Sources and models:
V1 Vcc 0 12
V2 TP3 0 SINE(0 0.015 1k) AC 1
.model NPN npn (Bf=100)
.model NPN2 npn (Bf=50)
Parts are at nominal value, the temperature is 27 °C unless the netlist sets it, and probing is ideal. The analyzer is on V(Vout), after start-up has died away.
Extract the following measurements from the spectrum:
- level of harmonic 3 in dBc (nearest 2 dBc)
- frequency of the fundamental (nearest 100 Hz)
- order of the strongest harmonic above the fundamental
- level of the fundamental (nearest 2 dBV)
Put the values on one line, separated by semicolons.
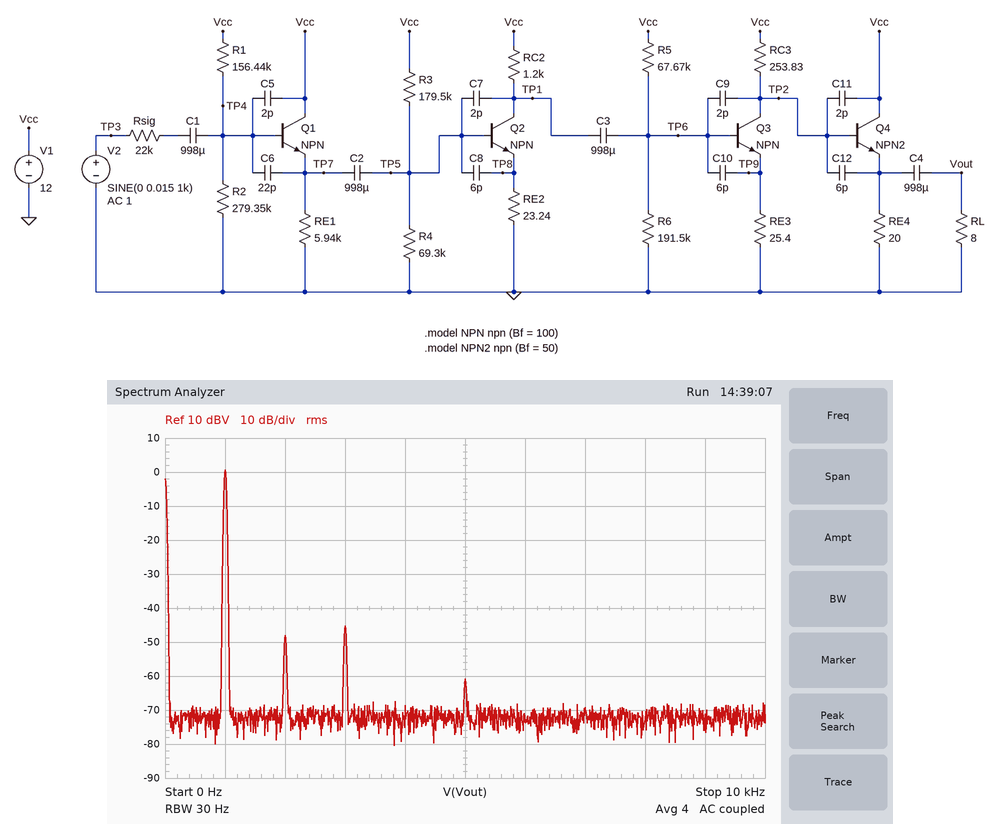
-46 dBc; 1.0 kHz; 3; 0 dBV
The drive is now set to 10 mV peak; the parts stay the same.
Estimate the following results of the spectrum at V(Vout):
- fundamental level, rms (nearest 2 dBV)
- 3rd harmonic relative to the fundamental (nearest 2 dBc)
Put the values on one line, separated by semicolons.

-2 dBV; -56 dBc
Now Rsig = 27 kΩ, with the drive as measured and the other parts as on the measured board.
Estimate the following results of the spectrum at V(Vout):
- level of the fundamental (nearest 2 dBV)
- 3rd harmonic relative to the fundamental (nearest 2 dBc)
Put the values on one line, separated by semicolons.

0 dBV; -48 dBc
